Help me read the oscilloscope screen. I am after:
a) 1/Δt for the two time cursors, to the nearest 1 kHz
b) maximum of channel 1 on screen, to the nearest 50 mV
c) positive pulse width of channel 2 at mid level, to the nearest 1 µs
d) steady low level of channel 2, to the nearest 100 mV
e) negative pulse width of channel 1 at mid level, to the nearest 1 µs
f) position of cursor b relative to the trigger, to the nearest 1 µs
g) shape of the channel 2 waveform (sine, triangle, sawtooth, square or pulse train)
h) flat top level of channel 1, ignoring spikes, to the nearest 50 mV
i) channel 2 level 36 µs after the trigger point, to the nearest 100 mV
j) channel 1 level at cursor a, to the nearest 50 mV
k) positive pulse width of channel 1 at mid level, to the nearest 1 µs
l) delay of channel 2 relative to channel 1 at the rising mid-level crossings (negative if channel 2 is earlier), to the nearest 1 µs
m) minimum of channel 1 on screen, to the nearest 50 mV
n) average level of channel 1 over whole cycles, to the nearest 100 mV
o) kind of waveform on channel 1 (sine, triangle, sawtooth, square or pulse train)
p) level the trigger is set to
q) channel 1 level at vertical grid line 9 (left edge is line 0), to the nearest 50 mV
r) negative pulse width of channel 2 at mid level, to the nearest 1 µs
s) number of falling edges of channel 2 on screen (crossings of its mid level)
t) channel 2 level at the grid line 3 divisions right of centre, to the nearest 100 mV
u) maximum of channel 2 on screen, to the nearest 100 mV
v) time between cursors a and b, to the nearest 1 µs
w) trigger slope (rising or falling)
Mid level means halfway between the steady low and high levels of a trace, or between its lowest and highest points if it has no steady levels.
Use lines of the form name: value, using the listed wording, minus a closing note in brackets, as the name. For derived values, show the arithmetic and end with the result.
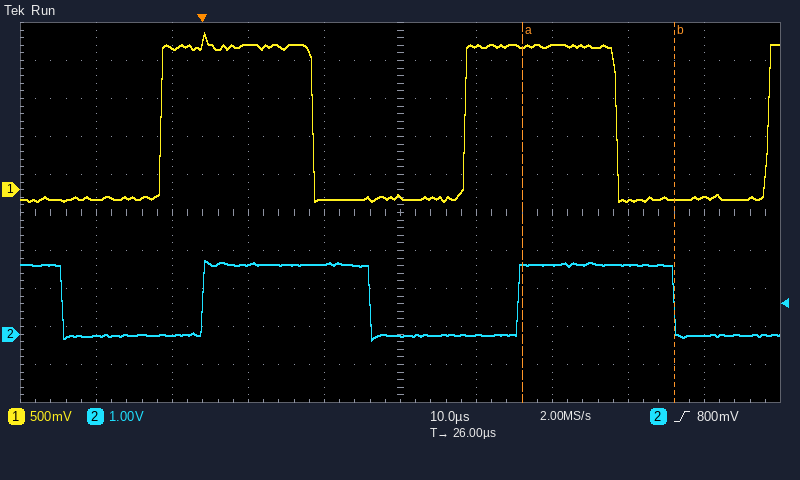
1/Δt for the two time cursors, to the nearest 1 kHz: 1 / 20 µs ≈ 50 kHz
maximum of channel 1 on screen, to the nearest 50 mV: 2.05 V
positive pulse width of channel 2 at mid level, to the nearest 1 µs: 21 µs
steady low level of channel 2, to the nearest 100 mV: 0.0 V
negative pulse width of channel 1 at mid level, to the nearest 1 µs: 20 µs
position of cursor b relative to the trigger, to the nearest 1 µs: +62 µs
shape of the channel 2 waveform: square
flat top level of channel 1, ignoring spikes, to the nearest 50 mV: 1.90 V
channel 2 level 36 µs after the trigger point, to the nearest 100 mV: 0.0 V
channel 1 level at cursor a, to the nearest 50 mV: 1.90 V
positive pulse width of channel 1 at mid level, to the nearest 1 µs: 20 µs
delay of channel 2 relative to channel 1 at the rising mid-level crossings (negative if channel 2 is earlier), to the nearest 1 µs: +6 µs
minimum of channel 1 on screen, to the nearest 50 mV: -150 mV
average level of channel 1 over whole cycles, to the nearest 100 mV: -150 mV + 0.5 × (1.90 V − (-150 mV)) ≈ 875 mV, so 900 mV to the nearest 100 mV
kind of waveform on channel 1: square
level the trigger is set to: 800 mV
channel 1 level at vertical grid line 9 (left edge is line 0), to the nearest 50 mV: -100 mV
negative pulse width of channel 2 at mid level, to the nearest 1 µs: 19 µs
number of falling edges of channel 2 on screen: 3
channel 2 level at the grid line 3 divisions right of centre, to the nearest 100 mV: 1.8 V
maximum of channel 2 on screen, to the nearest 100 mV: 1.9 V
time between cursors a and b, to the nearest 1 µs: 20 µs
trigger slope: rising
